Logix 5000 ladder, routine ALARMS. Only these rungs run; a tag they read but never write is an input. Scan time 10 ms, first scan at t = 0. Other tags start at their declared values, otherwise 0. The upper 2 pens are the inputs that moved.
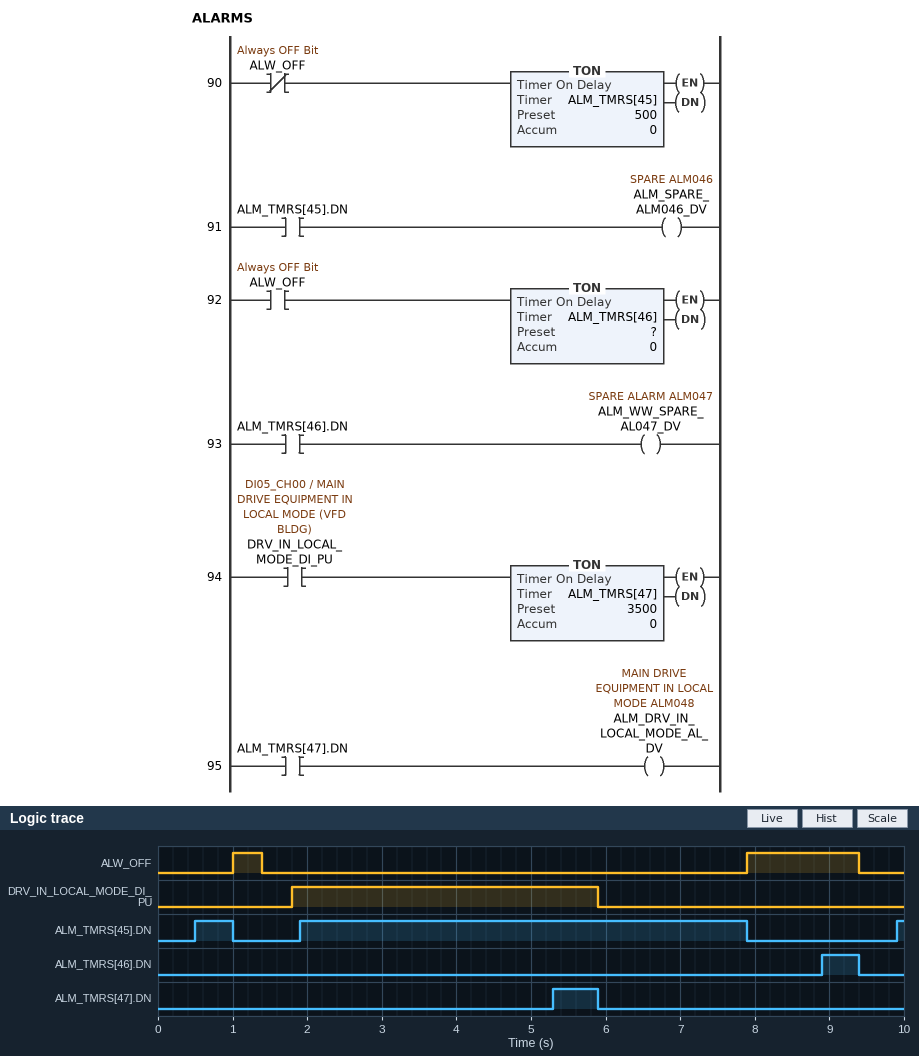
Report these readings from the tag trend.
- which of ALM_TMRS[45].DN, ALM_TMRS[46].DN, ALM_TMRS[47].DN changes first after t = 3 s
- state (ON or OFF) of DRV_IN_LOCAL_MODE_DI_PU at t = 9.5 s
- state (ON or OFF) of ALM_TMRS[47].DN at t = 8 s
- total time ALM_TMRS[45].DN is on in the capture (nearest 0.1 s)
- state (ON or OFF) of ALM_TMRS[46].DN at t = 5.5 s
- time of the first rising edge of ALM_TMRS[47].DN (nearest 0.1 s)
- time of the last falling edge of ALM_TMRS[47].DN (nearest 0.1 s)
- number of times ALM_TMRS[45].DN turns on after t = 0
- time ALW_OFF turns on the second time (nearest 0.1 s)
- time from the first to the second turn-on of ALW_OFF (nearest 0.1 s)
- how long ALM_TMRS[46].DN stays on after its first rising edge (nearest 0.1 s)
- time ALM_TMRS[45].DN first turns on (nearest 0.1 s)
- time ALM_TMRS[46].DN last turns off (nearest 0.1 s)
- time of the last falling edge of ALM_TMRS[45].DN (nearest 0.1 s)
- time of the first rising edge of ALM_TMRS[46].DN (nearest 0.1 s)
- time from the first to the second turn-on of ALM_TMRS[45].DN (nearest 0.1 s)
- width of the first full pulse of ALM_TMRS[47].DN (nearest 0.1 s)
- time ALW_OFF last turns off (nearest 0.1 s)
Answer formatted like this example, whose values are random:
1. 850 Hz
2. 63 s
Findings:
1. ALM_TMRS[47].DN
2. OFF
3. OFF
4. 6.6 s
5. OFF
6. 5.3 s
7. 5.9 s
8. 3
9. 7.9 s
10. 6.9 s
11. 0.5 s
12. 0.5 s
13. 9.4 s
14. 7.9 s
15. 8.9 s
16. 1.4 s
17. 0.6 s
18. 9.4 s
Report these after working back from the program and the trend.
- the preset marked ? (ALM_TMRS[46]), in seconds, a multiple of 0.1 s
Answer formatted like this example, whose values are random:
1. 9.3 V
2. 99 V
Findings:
1. 1.0 s
